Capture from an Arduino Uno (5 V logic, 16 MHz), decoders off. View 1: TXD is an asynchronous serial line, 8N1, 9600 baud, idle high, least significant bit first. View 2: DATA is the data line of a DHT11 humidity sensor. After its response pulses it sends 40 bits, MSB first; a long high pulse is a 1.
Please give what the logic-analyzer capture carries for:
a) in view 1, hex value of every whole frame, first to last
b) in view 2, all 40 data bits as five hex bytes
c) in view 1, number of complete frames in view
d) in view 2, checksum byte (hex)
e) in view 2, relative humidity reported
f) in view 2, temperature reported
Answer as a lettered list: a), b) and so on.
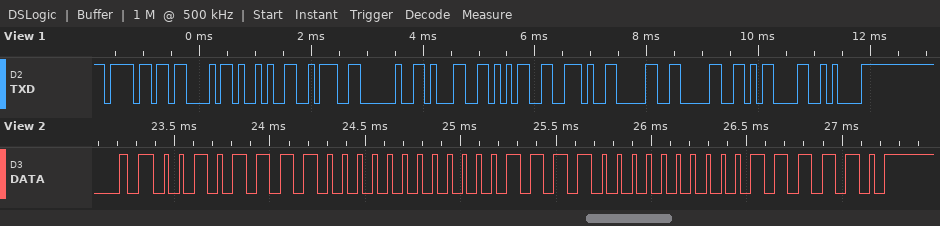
a) 6F 43 29 3A 20 31 35 2E 30 30 0D 0A
b) 2F 00 0F 00 3E
c) 12
d) 0x3E
e) 47 %
f) 15.0 °C
